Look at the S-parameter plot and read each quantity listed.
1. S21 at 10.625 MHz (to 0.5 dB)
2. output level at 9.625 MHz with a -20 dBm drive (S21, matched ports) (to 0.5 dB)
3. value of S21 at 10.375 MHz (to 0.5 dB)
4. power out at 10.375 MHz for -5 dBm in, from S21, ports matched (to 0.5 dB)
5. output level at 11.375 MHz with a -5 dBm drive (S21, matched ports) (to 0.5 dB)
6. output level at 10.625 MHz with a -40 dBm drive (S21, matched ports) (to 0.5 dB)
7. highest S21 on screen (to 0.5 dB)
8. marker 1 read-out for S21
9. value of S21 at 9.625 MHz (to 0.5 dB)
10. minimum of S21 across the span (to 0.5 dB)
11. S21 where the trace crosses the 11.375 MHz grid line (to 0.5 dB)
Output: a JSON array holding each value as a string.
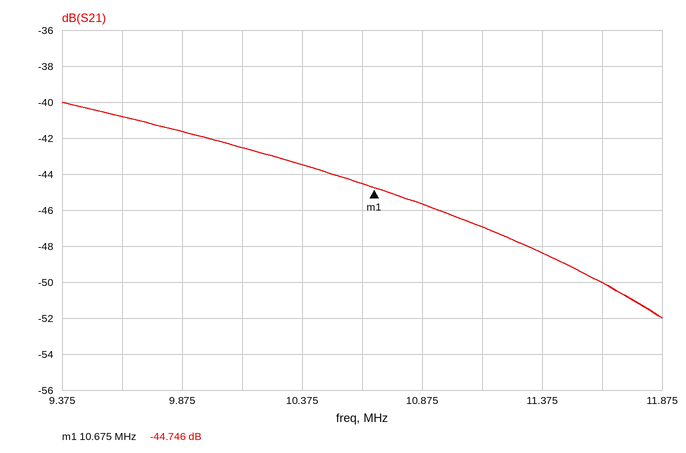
["-44.5 dB", "-61.0 dBm", "-43.5 dB", "-48.5 dBm", "-53.5 dBm", "-84.5 dBm", "-40.0 dB", "-44.746 dB", "-41.0 dB", "-52.0 dB", "-48.5 dB"]
